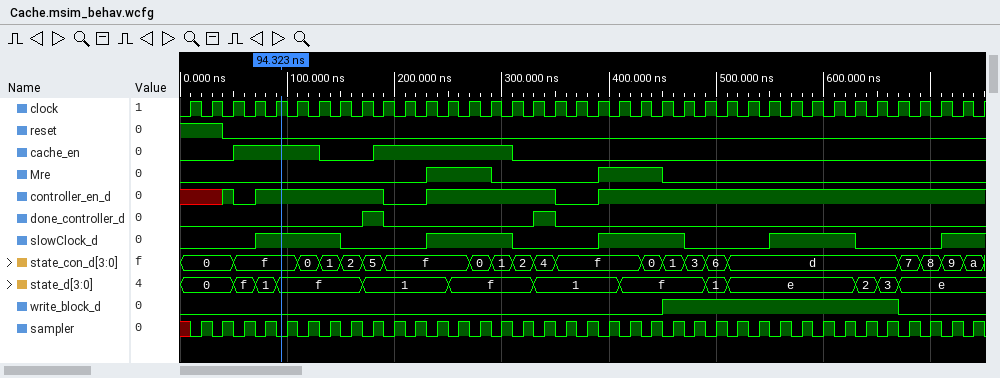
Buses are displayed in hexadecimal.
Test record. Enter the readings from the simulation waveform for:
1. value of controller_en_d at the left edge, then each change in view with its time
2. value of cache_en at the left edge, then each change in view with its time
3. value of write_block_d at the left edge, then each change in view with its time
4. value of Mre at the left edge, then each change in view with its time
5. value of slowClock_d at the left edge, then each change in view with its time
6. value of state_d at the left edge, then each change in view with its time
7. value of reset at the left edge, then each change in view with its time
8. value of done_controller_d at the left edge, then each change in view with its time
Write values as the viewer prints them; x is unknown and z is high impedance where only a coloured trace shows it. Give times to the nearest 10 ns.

x, 1 at 40 ns, 0 at 50 ns, 1 at 70 ns, 0 at 190 ns, 1 at 230 ns, 0 at 350 ns, 1 at 390 ns
0, 1 at 50 ns, 0 at 130 ns, 1 at 180 ns, 0 at 310 ns
0, 1 at 450 ns, 0 at 670 ns
0, 1 at 230 ns, 0 at 290 ns, 1 at 390 ns, 0 at 450 ns
0, 1 at 70 ns, 0 at 150 ns, 1 at 230 ns, 0 at 310 ns, 1 at 390 ns, 0 at 470 ns, 1 at 550 ns, 0 at 630 ns, 1 at 710 ns
0, f at 50 ns, 1 at 70 ns, f at 90 ns, 1 at 170 ns, f at 250 ns, 1 at 330 ns, f at 410 ns, 1 at 490 ns, e at 510 ns, 2 at 630 ns, 3 at 650 ns, e at 670 ns
1, 0 at 40 ns
0, 1 at 170 ns, 0 at 190 ns, 1 at 330 ns, 0 at 350 ns
